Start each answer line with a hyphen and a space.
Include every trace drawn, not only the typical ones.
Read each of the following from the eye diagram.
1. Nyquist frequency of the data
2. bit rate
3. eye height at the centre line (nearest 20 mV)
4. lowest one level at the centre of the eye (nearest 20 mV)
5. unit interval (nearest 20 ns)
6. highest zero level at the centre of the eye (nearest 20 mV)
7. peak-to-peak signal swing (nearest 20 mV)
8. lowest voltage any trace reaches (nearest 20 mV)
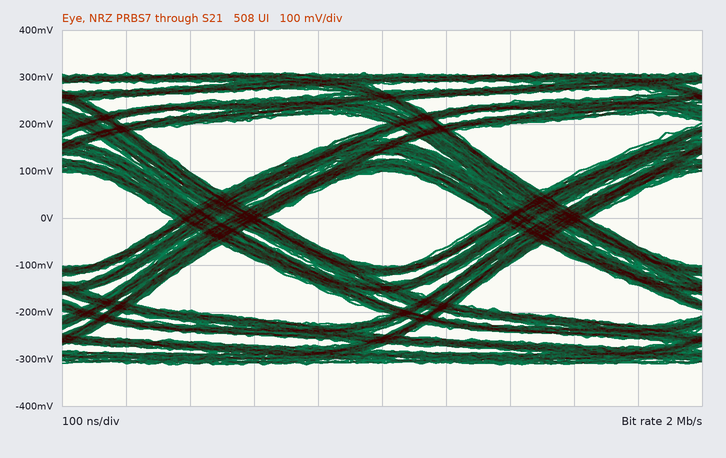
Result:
- 1 MHz
- 2 Mb/s
- 200 mV
- 100 mV
- 500 ns
- -100 mV
- 620 mV
- -320 mV
